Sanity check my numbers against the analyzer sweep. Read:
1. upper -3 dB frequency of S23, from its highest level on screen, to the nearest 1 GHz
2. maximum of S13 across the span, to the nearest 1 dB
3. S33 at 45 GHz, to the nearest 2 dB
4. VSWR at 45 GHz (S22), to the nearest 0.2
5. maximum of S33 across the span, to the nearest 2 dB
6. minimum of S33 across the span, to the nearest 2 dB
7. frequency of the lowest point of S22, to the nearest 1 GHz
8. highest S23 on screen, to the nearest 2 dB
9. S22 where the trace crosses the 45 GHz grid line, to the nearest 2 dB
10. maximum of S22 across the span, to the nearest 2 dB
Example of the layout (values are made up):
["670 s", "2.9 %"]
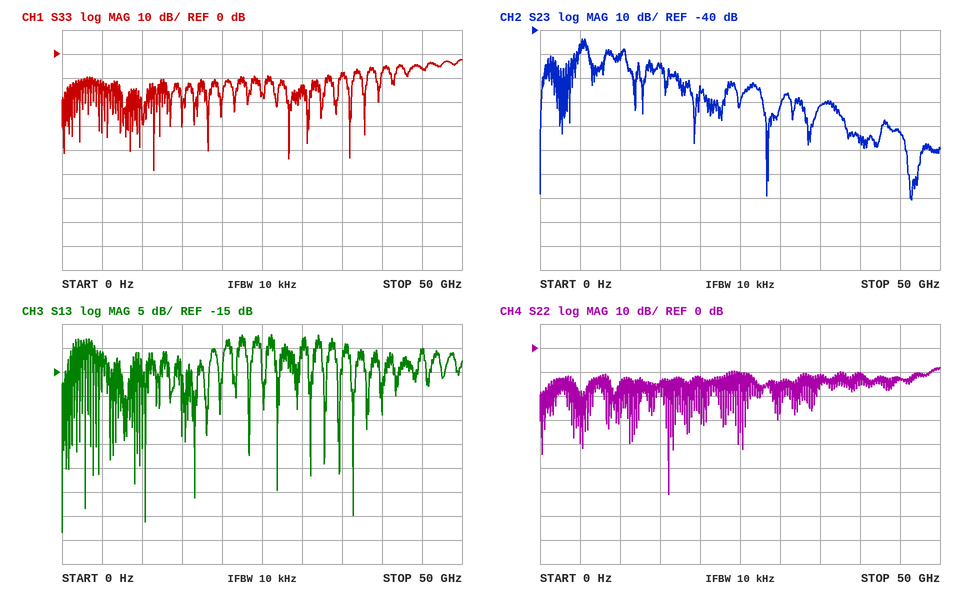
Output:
["6 GHz", "-7 dB", "-6 dB", "1.6", "-2 dB", "-48 dB", "16 GHz", "-44 dB", "-12 dB", "-8 dB"]
